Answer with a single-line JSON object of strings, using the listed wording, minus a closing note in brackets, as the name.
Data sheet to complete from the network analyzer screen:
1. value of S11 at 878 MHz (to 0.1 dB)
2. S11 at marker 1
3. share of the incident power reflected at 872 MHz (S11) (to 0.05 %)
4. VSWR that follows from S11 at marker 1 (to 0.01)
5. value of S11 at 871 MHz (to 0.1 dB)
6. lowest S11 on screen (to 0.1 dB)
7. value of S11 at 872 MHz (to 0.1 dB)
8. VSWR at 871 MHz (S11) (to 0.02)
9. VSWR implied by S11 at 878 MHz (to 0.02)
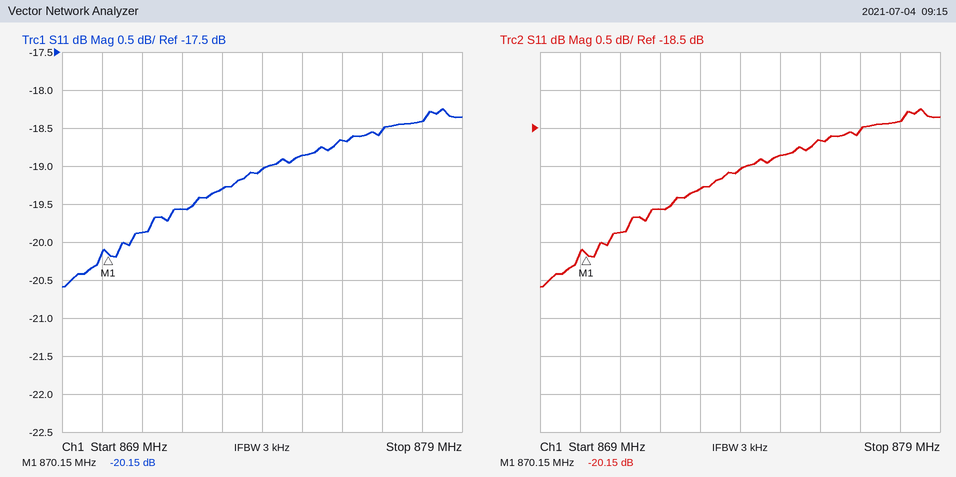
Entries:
{"value of S11 at 878 MHz": "-18.4 dB", "S11 at marker 1": "-20.15 dB", "share of the incident power reflected at 872 MHz (S11)": "1.10 %", "VSWR that follows from S11 at marker 1": "1.22", "value of S11 at 871 MHz": "-19.9 dB", "lowest S11 on screen": "-20.6 dB", "value of S11 at 872 MHz": "-19.6 dB", "VSWR at 871 MHz (S11)": "1.22", "VSWR implied by S11 at 878 MHz": "1.28"}
